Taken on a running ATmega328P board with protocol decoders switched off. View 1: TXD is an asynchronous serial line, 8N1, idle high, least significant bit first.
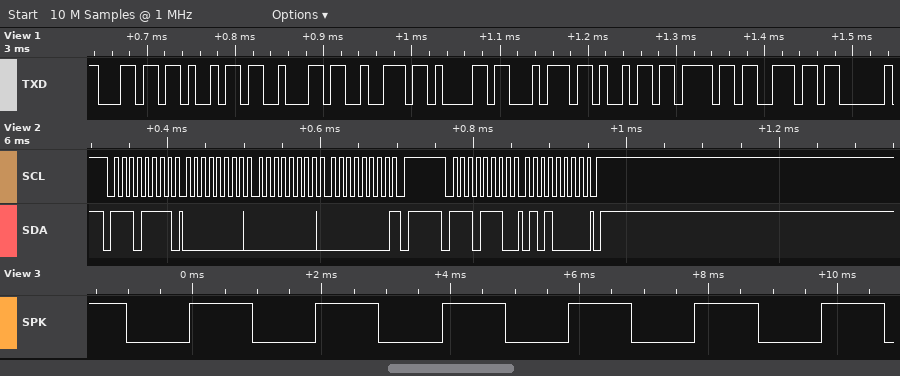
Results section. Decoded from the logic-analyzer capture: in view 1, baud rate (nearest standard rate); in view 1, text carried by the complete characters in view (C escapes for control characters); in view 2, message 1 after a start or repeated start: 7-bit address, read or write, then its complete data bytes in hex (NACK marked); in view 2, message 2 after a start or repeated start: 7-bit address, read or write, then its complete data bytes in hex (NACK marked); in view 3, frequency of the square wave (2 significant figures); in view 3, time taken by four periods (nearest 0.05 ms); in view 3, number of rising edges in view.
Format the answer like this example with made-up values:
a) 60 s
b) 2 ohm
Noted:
a) 115200 baud
b) "libration"
c) 0x77 read: 00 00 00 NACK
d) 0x77 write: 50
e) 510 Hz
f) 7.85 ms
g) 6
